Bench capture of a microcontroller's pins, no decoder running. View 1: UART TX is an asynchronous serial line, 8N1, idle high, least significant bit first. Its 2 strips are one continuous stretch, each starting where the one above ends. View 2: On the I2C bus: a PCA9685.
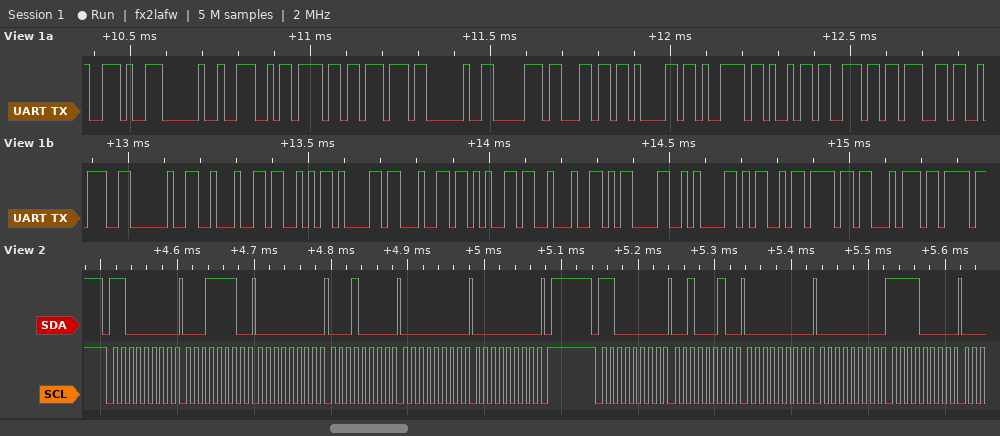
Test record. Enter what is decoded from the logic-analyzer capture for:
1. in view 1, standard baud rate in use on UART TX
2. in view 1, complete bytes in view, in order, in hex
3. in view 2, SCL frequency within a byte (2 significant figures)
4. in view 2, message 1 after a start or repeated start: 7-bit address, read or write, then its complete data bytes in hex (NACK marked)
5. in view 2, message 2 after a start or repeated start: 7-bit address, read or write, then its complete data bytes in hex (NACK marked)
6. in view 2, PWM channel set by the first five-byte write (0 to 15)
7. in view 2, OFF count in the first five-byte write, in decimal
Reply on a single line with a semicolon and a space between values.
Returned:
57600 baud; 2E 20 4E 6F 77 20 70 6C 61 79 69 6E 67 3A 20 22 53 61 64 65 22 0D 0A 4D 6F 74; 100 kHz; 0x60 write: 1E 00 10 00 00; 0x60 write: 22 00 00 F0; 6; 0
